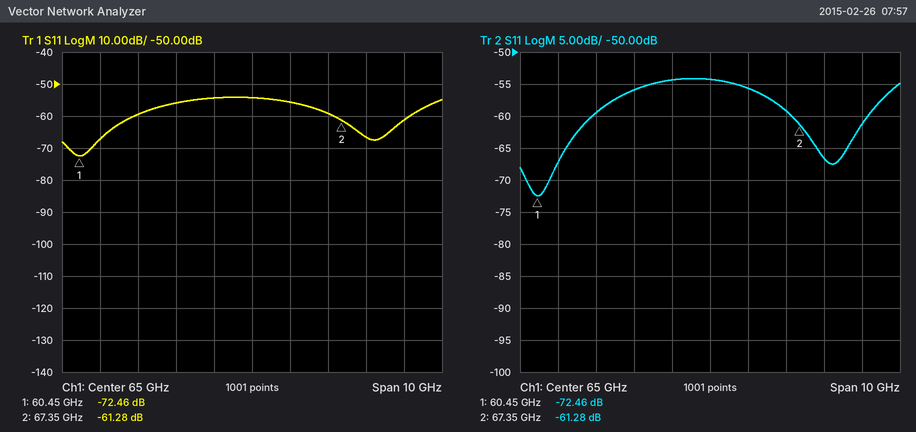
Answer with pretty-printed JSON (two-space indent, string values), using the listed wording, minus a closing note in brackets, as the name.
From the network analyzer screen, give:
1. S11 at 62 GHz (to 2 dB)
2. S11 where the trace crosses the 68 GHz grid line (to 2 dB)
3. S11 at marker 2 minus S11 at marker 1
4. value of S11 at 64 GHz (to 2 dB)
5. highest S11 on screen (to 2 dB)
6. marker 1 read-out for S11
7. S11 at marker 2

{
  "S11 at 62 GHz": "-60 dB",
  "S11 where the trace crosses the 68 GHz grid line": "-66 dB",
  "S11 at marker 2 minus S11 at marker 1": "11.18 dB",
  "value of S11 at 64 GHz": "-54 dB",
  "highest S11 on screen": "-54 dB",
  "marker 1 read-out for S11": "-72.46 dB",
  "S11 at marker 2": "-61.28 dB"
}
